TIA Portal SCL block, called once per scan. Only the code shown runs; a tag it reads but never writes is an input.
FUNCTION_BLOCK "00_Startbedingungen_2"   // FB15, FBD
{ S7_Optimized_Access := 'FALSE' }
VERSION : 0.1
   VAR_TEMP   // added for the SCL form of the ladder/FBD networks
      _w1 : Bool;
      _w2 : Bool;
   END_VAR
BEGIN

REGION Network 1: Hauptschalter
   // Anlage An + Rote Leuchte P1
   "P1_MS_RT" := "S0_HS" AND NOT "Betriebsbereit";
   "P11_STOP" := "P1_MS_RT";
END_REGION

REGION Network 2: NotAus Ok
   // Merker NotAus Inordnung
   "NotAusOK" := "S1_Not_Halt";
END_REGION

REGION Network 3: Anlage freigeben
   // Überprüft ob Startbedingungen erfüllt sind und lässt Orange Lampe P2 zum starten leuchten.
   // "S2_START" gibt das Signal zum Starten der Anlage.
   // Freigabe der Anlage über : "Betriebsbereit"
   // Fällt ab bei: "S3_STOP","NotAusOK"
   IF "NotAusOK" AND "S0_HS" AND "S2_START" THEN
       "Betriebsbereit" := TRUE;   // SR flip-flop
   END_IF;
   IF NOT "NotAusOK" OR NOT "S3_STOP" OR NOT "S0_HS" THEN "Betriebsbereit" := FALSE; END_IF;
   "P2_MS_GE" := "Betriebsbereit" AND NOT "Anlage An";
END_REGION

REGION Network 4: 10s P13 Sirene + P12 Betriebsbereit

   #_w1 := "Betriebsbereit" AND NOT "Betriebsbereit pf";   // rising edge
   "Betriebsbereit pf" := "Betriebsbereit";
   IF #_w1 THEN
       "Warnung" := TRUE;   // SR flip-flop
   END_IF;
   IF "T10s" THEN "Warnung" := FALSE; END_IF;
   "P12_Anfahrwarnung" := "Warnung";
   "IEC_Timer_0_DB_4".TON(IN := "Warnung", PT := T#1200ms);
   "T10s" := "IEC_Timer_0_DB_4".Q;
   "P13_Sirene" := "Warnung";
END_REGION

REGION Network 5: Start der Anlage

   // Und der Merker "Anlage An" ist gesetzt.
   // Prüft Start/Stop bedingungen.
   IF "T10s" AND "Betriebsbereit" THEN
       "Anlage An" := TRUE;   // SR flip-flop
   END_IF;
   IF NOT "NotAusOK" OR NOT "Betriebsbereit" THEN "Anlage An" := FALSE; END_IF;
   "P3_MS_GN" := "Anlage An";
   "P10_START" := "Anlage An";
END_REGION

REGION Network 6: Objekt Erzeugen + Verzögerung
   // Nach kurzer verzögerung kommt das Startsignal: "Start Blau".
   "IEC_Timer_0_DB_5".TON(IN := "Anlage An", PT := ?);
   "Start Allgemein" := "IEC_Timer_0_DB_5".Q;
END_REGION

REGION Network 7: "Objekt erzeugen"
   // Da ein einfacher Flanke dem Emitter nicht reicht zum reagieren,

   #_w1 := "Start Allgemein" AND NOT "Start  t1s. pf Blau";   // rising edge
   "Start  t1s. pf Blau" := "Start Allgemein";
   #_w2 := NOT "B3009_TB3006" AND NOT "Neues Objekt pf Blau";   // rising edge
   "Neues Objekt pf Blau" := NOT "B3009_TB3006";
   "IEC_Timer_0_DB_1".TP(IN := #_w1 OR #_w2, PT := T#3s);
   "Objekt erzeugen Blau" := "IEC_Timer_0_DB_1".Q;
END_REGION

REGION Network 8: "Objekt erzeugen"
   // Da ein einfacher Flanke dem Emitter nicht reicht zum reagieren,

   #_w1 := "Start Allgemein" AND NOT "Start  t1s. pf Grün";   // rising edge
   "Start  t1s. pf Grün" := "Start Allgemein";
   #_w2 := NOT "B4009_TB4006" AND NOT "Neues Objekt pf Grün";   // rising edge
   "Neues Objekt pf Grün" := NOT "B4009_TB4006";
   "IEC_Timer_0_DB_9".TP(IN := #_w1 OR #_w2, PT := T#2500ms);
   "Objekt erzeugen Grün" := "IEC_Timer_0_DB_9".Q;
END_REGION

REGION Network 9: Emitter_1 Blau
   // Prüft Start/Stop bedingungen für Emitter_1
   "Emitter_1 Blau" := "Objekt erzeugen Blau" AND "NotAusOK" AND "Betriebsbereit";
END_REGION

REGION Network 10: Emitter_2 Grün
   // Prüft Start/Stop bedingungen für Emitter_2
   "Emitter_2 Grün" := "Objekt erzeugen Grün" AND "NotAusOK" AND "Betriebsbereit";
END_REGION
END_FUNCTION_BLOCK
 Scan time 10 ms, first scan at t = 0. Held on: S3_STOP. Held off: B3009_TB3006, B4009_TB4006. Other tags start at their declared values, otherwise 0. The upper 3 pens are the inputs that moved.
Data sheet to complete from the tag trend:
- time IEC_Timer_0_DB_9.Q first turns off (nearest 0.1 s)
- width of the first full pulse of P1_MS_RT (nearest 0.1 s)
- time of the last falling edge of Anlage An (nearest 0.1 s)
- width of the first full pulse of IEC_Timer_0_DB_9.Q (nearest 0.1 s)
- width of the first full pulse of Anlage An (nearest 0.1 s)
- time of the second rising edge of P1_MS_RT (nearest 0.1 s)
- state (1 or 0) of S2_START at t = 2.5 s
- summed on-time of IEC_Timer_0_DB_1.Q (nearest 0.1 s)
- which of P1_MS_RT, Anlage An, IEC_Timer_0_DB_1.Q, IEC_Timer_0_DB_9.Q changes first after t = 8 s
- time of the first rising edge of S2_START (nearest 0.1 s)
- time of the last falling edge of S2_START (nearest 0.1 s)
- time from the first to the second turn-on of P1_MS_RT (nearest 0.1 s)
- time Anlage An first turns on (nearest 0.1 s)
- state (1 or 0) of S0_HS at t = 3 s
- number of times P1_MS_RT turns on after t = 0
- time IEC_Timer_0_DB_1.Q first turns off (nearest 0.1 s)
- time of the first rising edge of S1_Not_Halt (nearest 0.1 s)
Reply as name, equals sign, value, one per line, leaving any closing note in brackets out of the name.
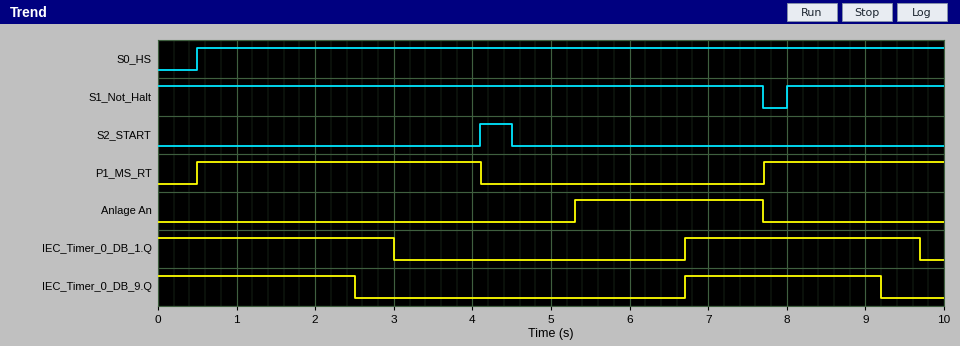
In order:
time IEC_Timer_0_DB_9.Q first turns off = 2.5 s
width of the first full pulse of P1_MS_RT = 3.6 s
time of the last falling edge of Anlage An = 7.7 s
width of the first full pulse of IEC_Timer_0_DB_9.Q = 2.5 s
width of the first full pulse of Anlage An = 2.4 s
time of the second rising edge of P1_MS_RT = 7.7 s
state (1 or 0) of S2_START at t = 2.5 s = 0
summed on-time of IEC_Timer_0_DB_1.Q = 6.0 s
which of P1_MS_RT, Anlage An, IEC_Timer_0_DB_1.Q, IEC_Timer_0_DB_9.Q changes first after t = 8 s = IEC_Timer_0_DB_9.Q
time of the first rising edge of S2_START = 4.1 s
time of the last falling edge of S2_START = 4.5 s
time from the first to the second turn-on of P1_MS_RT = 7.2 s
time Anlage An first turns on = 5.3 s
state (1 or 0) of S0_HS at t = 3 s = 1
number of times P1_MS_RT turns on after t = 0 = 2
time IEC_Timer_0_DB_1.Q first turns off = 3.0 s
time of the first rising edge of S1_Not_Halt = 8.0 s
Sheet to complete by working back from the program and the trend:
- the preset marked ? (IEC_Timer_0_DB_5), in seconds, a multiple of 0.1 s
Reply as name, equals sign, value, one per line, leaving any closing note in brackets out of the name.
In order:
the preset marked ? (IEC_Timer_0_DB_5), in seconds, a multiple of 0.1 s = 1.4 s
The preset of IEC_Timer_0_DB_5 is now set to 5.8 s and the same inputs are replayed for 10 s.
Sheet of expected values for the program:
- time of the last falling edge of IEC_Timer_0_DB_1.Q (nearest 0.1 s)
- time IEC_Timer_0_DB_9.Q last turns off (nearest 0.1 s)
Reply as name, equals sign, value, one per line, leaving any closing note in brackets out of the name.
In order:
time of the last falling edge of IEC_Timer_0_DB_1.Q = 3.0 s
time IEC_Timer_0_DB_9.Q last turns off = 2.5 s
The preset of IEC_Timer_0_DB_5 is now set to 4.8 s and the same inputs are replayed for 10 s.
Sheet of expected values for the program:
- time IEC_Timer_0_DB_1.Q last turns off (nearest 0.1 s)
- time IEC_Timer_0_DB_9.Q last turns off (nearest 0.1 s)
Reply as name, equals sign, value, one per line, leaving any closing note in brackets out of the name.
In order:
time IEC_Timer_0_DB_1.Q last turns off = 3.0 s
time IEC_Timer_0_DB_9.Q last turns off = 2.5 s
